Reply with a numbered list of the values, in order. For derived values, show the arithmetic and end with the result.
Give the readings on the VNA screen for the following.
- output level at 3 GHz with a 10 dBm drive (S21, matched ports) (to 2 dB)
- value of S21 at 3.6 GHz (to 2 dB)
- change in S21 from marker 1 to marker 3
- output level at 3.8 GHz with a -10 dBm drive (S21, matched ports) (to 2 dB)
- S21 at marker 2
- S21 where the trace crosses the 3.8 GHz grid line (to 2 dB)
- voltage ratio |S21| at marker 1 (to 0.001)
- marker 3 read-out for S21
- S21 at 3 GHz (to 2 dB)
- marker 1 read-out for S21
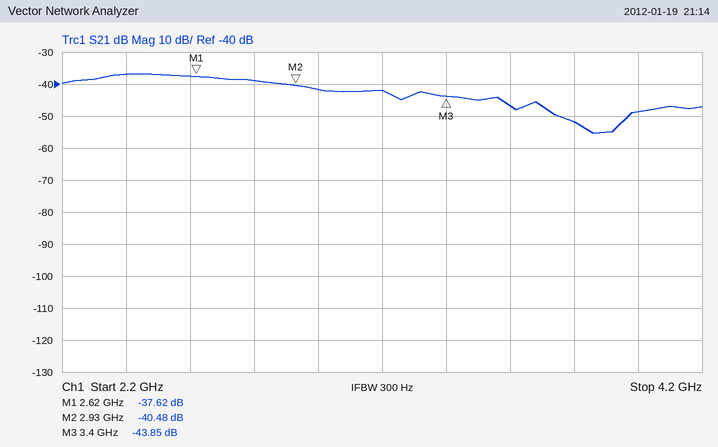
1. 10 dBm + (-42 dB) = -32 dBm
2. -46 dB
3. -43.85 − (-37.62) = -6.23 dB
4. -10 dBm + (-52 dB) = -62 dBm
5. -40.48 dB
6. -52 dB
7. 10^(-37.62/20) ≈ 0.013
8. -43.85 dB
9. -42 dB
10. -37.62 dB
